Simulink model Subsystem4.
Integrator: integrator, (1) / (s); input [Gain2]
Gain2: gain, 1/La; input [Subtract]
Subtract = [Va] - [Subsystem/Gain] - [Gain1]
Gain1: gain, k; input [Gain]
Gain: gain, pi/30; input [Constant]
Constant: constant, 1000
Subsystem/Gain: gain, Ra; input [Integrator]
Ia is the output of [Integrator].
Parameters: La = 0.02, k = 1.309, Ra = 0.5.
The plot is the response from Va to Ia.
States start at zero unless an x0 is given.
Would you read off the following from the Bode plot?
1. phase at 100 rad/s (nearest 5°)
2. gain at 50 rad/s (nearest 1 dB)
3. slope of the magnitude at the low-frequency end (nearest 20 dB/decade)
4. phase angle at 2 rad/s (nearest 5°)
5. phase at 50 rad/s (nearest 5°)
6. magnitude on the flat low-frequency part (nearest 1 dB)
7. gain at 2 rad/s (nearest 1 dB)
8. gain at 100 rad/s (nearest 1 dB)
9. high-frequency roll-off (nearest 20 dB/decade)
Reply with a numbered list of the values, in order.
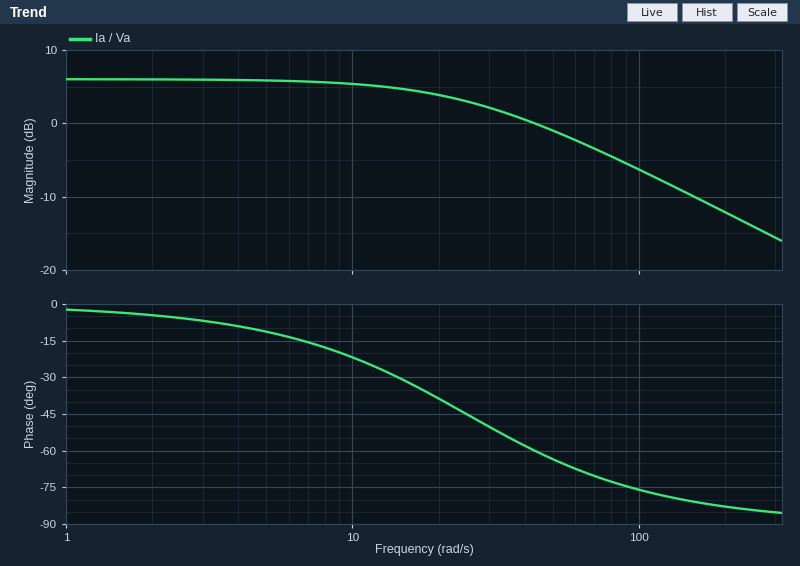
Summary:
1. -75°
2. -1 dB
3. 0 dB/decade
4. -5°
5. -65°
6. 6 dB
7. 6 dB
8. -6 dB
9. -20 dB/decade
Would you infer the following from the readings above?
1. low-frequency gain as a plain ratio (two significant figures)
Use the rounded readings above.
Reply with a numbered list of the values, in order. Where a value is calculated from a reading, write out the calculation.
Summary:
1. 10^(6 / 20) = 2.0
